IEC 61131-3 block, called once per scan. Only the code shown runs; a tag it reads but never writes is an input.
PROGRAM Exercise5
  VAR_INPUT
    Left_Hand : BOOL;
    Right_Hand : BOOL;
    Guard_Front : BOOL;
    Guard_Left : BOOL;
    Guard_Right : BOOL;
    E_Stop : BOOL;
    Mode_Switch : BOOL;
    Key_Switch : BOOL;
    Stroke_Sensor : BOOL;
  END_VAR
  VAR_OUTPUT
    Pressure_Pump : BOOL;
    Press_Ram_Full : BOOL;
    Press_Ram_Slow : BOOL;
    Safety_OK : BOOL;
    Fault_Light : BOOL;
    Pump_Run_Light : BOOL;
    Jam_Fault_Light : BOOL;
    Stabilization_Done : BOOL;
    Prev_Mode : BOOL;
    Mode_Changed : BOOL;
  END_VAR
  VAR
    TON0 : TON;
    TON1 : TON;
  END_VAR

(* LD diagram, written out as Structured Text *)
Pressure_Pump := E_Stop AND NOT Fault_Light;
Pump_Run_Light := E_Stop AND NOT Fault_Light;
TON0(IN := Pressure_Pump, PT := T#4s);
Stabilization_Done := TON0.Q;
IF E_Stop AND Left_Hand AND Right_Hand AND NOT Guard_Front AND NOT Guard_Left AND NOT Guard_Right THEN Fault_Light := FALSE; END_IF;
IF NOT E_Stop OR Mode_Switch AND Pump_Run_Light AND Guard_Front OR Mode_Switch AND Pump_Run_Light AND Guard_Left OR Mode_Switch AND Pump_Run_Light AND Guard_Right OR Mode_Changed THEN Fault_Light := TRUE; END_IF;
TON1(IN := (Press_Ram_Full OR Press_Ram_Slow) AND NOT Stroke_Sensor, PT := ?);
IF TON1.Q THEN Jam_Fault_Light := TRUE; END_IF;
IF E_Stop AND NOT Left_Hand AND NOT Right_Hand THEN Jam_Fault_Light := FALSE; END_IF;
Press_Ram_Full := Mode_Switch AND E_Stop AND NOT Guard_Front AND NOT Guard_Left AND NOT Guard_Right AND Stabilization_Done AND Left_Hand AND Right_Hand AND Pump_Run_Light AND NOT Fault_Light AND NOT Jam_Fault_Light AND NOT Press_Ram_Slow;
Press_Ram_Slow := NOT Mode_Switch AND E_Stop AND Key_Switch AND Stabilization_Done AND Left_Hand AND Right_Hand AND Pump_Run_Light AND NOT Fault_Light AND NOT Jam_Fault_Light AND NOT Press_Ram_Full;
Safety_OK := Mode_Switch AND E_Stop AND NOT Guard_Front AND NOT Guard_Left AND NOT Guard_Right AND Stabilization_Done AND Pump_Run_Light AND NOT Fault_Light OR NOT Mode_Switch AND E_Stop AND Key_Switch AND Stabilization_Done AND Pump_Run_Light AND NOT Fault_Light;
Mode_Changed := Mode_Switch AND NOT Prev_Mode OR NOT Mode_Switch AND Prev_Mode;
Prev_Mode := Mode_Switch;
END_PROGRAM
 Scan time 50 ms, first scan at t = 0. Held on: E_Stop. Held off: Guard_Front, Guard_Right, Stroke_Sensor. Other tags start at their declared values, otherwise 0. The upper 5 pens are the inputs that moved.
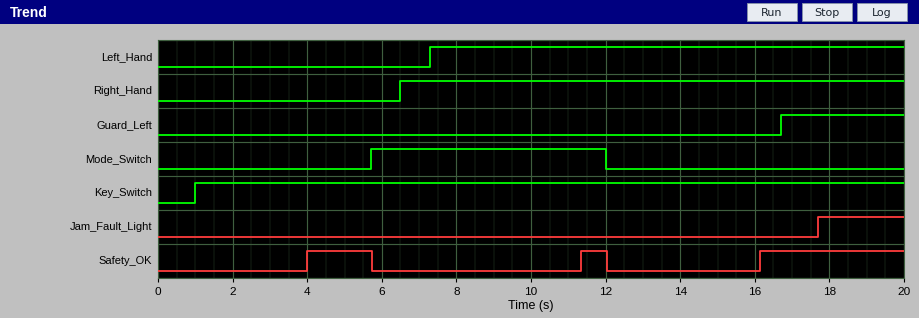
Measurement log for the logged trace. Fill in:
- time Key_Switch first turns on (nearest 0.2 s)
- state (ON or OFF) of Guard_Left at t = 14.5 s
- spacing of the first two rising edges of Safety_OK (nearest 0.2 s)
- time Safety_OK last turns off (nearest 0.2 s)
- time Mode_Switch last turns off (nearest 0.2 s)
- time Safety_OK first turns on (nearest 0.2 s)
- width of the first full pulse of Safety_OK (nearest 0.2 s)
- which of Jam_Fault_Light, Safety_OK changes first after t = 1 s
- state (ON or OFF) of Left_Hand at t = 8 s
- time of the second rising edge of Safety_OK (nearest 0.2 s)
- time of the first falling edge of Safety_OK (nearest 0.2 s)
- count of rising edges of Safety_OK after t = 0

1.0 s
OFF
7.4 s
12.0 s
12.0 s
4.0 s
1.8 s
Safety_OK
ON
11.4 s
5.8 s
3
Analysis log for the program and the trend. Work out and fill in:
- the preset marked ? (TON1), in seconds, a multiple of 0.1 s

1.5 s
